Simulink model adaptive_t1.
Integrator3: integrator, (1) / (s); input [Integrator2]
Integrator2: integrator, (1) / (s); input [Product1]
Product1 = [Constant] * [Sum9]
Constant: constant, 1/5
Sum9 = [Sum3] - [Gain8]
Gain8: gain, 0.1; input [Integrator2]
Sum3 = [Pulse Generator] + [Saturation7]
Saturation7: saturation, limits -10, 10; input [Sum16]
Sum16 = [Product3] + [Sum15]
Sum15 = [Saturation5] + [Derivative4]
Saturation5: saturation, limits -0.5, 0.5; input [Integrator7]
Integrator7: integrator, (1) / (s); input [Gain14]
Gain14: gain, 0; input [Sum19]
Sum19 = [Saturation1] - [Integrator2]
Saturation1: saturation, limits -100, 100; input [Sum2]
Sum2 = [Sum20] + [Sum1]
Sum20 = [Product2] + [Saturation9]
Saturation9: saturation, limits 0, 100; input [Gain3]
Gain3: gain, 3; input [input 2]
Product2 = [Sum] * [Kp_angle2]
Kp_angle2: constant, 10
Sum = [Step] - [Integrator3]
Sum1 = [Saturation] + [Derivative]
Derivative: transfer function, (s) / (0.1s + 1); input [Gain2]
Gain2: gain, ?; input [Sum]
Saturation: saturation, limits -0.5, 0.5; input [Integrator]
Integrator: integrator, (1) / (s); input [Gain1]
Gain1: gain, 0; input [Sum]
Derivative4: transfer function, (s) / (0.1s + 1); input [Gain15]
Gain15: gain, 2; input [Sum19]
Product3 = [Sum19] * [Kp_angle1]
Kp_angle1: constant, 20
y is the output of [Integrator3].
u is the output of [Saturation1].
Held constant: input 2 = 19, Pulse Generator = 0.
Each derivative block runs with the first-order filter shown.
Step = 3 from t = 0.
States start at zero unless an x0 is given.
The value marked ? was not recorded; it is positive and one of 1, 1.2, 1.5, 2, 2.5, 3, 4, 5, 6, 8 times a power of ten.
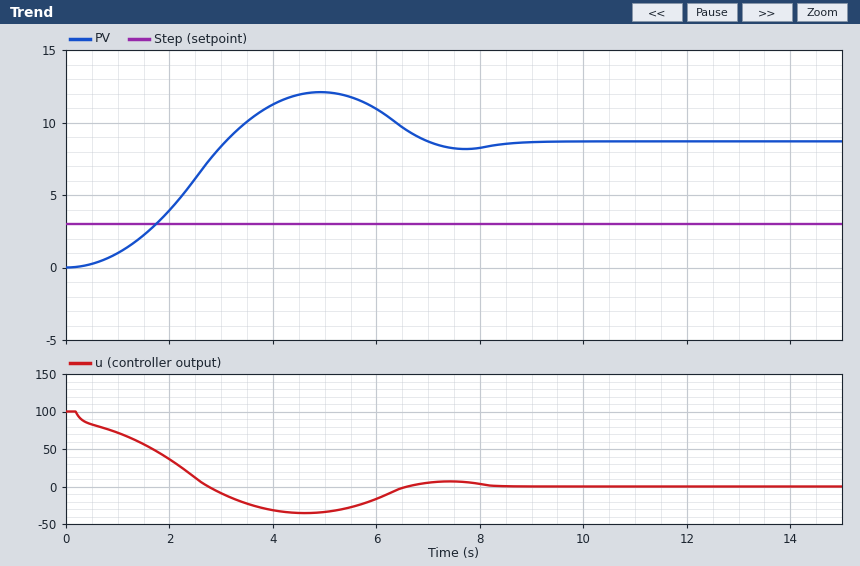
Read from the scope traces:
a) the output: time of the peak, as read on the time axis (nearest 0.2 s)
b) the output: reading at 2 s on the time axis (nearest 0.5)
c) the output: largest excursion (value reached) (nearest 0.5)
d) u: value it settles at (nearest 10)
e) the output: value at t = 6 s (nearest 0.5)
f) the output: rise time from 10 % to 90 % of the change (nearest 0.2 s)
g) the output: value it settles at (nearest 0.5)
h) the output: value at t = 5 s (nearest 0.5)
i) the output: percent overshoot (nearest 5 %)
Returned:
5.0 s
4.0
12.0
0
11.0
2.0 s
8.5
12.0
40 %
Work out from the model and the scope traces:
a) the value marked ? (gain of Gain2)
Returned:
3
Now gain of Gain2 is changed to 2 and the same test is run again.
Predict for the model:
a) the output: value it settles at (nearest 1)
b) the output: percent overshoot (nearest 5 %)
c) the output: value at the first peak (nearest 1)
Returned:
9
50 %
13
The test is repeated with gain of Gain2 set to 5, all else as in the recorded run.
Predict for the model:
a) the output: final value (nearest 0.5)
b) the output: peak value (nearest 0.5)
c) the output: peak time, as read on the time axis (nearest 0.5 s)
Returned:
8.5
10.5
4.5 s
